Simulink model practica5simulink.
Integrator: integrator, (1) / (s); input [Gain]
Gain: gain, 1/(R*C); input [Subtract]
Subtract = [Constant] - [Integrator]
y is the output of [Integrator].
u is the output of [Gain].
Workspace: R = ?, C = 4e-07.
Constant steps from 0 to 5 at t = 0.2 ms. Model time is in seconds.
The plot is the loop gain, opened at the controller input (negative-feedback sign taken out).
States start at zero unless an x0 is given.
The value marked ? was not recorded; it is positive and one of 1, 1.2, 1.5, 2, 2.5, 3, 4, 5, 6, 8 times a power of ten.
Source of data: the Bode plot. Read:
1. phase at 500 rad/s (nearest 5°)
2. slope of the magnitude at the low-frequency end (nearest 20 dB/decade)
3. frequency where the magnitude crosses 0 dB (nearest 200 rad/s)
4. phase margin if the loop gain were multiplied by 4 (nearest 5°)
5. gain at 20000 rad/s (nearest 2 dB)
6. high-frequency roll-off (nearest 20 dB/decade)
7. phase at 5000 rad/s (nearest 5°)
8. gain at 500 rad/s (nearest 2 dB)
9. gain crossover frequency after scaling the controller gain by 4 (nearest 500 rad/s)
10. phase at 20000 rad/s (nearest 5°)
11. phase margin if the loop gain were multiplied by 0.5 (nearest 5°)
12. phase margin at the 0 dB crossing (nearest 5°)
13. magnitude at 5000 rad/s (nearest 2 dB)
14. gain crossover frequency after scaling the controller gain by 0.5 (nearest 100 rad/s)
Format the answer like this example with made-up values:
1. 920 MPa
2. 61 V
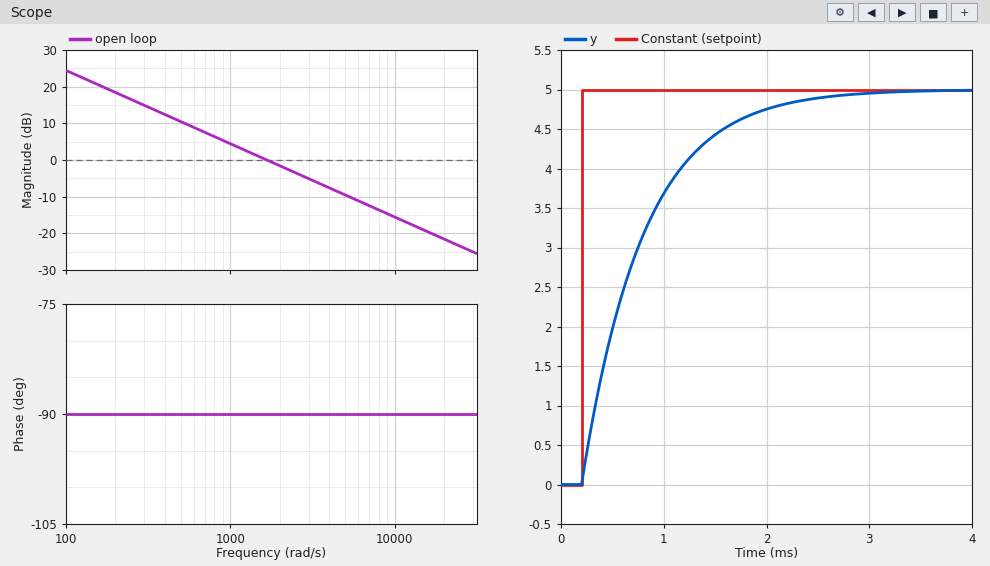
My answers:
1. -90°
2. -20 dB/decade
3. 1600 rad/s
4. 90°
5. -22 dB
6. -20 dB/decade
7. -90°
8. 10 dB
9. 6500 rad/s
10. -90°
11. 90°
12. 90°
13. -10 dB
14. 800 rad/s
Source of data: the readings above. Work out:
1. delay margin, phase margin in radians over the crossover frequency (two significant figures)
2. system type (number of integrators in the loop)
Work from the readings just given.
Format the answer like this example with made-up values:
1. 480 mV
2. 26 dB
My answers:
1. 0.00098 s
2. 1
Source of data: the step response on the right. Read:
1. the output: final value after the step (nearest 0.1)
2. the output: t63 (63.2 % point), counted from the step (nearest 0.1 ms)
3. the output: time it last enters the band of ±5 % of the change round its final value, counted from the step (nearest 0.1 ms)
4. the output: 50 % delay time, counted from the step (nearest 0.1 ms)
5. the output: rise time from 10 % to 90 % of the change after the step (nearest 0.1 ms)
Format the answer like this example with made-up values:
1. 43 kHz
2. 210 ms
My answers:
1. 5.0
2. 0.6 ms
3. 1.8 ms
4. 0.4 ms
5. 1.3 ms
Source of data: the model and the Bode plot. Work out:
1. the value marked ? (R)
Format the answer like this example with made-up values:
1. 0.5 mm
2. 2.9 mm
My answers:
1. 1500
